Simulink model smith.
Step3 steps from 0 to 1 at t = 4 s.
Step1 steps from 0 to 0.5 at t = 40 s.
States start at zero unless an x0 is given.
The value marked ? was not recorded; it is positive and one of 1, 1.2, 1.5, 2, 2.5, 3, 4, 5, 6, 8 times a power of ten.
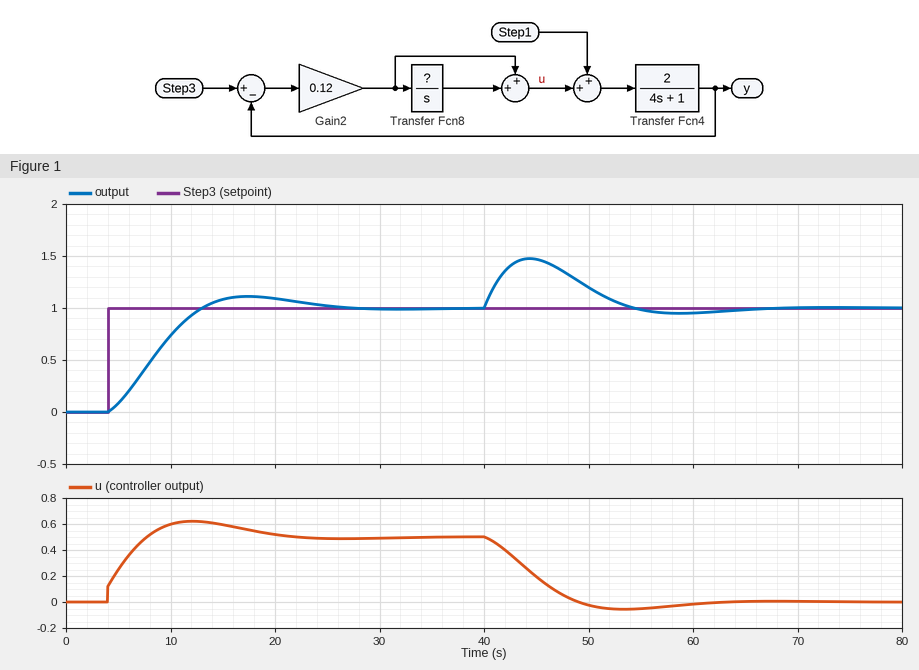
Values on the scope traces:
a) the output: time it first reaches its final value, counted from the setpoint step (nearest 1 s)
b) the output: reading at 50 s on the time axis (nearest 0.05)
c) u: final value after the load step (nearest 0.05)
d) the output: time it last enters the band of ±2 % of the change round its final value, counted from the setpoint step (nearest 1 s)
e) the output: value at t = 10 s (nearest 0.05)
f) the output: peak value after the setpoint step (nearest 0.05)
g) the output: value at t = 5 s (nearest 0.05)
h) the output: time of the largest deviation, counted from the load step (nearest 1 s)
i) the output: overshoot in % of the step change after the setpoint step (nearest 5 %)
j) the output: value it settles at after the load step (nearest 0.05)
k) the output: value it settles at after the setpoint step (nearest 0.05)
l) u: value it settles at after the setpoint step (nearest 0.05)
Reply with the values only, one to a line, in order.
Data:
9 s
1.20
0.00
21 s
0.75
1.10
0.10
4 s
10 %
1.00
1.00
0.50
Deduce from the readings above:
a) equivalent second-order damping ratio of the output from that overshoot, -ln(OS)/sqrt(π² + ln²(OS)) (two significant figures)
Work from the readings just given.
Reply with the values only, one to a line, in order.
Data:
0.59
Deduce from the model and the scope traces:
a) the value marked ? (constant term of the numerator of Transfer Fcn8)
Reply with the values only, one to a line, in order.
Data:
1.2
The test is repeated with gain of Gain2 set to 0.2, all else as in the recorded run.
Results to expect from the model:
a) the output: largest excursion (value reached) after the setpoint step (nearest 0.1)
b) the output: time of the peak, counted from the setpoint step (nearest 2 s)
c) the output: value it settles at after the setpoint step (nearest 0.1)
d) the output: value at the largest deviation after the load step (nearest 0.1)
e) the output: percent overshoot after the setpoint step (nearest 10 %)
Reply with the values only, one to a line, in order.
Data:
1.2
10 s
1.0
1.4
20 %
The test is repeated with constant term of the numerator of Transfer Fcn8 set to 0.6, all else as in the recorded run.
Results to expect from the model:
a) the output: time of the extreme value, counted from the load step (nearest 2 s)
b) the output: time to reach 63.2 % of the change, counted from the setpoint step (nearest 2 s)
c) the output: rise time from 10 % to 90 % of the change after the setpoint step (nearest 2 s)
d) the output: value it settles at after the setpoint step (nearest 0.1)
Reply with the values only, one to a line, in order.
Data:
6 s
8 s
12 s
1.0
